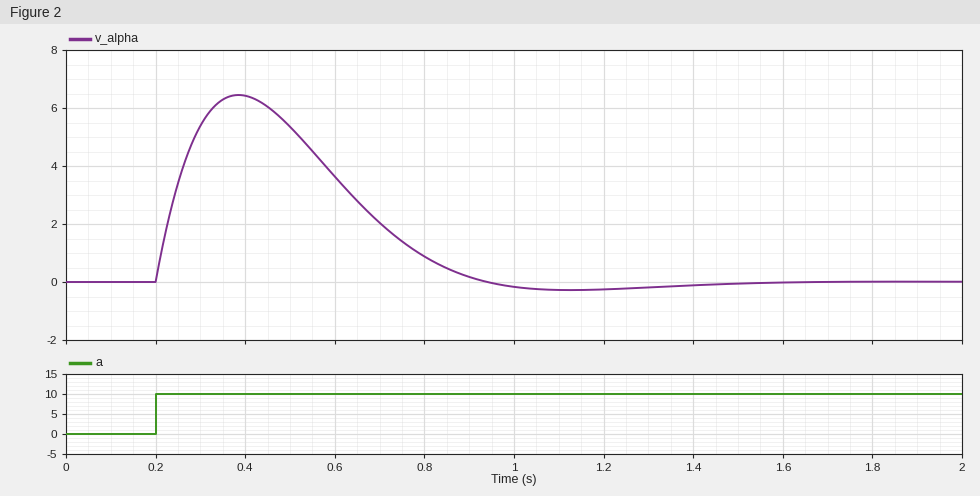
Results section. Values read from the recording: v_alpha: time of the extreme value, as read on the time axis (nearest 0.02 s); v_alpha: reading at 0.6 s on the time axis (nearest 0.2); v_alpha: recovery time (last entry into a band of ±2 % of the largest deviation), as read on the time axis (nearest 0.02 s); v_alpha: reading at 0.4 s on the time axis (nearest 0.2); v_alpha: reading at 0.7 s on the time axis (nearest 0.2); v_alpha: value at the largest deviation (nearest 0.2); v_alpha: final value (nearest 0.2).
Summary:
0.38 s
3.6
1.38 s
6.4
2.0
6.4
0.0
